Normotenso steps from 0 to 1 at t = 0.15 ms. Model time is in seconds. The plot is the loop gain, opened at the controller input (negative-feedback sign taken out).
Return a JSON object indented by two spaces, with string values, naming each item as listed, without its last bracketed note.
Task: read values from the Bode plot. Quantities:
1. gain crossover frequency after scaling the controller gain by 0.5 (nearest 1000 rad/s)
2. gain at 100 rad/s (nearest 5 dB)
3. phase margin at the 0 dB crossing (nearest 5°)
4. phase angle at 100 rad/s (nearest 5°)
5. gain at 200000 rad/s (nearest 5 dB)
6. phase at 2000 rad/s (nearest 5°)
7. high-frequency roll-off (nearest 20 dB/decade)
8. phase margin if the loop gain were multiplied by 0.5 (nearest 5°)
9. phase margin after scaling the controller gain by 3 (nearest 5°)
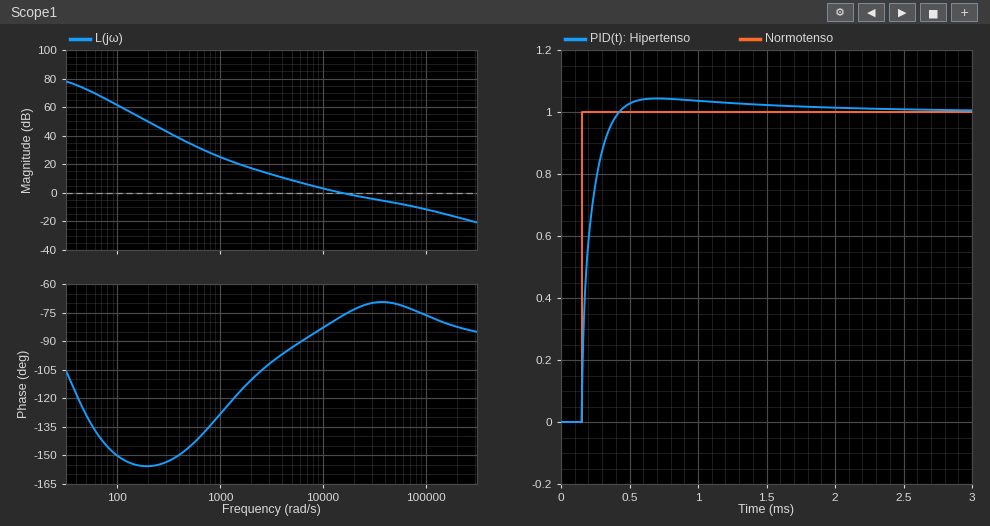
{
  "gain crossover frequency after scaling the controller gain by 0.5": "7000 rad/s",
  "gain at 100 rad/s": "60 dB",
  "phase margin at the 0 dB crossing": "105°",
  "phase angle at 100 rad/s": "-150°",
  "gain at 200000 rad/s": "-15 dB",
  "phase at 2000 rad/s": "-110°",
  "high-frequency roll-off": "-20 dB/decade",
  "phase margin if the loop gain were multiplied by 0.5": "90°",
  "phase margin after scaling the controller gain by 3": "105°"
}
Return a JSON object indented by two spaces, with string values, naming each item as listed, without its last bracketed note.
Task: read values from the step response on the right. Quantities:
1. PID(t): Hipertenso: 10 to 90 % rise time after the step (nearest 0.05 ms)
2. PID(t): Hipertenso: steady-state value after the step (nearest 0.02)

{
  "PID(t): Hipertenso: 10 to 90 % rise time after the step": "0.15 ms",
  "PID(t): Hipertenso: steady-state value after the step": "1.00"
}
